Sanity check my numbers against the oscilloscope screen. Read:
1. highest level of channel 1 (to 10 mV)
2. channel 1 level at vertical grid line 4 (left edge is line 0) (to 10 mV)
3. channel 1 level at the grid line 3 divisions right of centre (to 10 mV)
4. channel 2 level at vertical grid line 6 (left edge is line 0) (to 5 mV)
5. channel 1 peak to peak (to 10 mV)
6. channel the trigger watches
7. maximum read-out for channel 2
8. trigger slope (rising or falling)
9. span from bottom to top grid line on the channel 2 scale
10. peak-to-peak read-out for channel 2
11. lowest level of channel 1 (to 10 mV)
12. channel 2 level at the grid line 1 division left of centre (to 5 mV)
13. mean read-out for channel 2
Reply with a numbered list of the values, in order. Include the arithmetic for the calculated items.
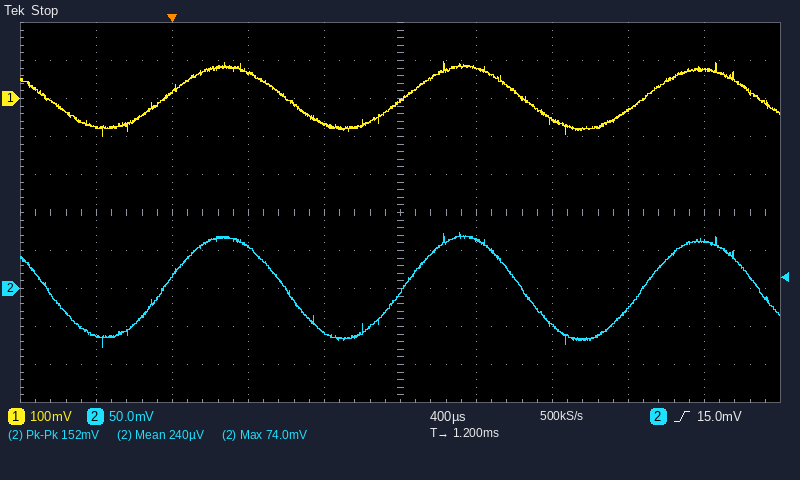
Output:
1. 100 mV
2. -70 mV
3. -30 mV
4. 65 mV
5. 100 mV − (-100 mV) = 200 mV
6. channel 2
7. 74.0 mV
8. rising
9. 500 mV
10. 152 mV
11. -100 mV
12. -60 mV
13. 240 µV
